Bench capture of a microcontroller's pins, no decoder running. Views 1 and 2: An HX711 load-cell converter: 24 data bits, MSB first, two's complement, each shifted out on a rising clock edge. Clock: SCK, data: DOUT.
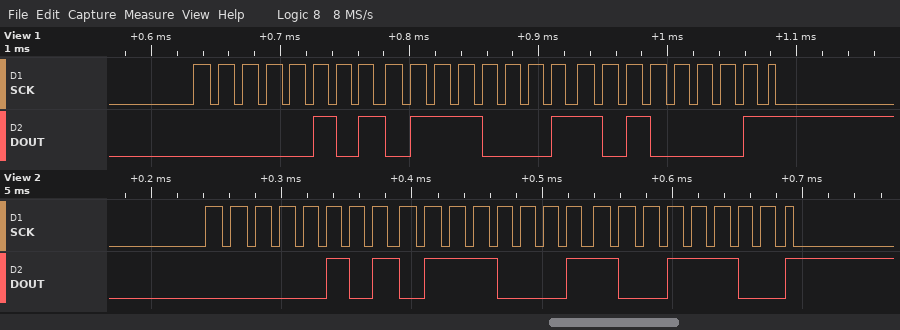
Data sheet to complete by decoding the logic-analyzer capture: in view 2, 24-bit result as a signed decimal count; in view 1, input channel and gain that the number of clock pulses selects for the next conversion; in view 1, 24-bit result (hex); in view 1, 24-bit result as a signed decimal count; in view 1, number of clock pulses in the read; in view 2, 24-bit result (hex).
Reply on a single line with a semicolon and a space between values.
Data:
356764; channel A, gain 128; 0x0571A1; 356769; 25; 0x05719C
